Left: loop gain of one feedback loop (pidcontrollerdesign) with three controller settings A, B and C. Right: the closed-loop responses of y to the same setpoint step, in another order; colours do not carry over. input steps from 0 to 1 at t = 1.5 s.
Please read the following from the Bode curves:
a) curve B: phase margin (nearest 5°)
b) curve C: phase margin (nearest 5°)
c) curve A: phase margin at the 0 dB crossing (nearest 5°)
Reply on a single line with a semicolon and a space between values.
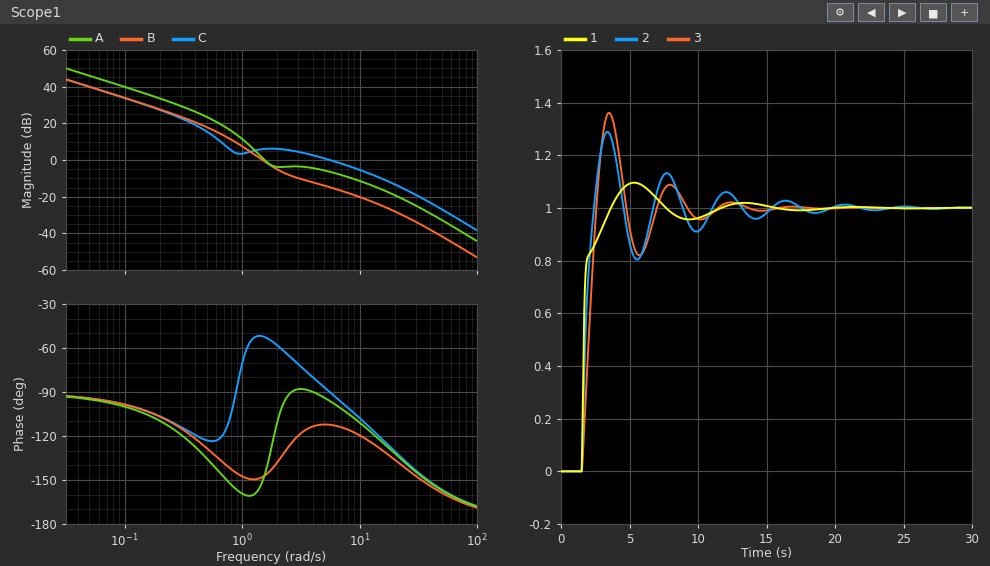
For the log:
30°; 90°; 35°
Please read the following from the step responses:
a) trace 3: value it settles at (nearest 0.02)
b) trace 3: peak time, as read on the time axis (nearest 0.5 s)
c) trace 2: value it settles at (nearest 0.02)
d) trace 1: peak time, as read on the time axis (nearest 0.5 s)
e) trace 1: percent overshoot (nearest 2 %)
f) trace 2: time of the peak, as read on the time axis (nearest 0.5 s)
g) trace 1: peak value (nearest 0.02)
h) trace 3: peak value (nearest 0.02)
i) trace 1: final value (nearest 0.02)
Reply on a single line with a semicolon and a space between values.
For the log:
1.00; 3.5 s; 1.00; 5.5 s; 10 %; 3.5 s; 1.10; 1.36; 1.00
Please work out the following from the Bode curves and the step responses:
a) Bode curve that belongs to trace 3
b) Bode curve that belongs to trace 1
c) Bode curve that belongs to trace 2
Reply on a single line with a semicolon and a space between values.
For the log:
B; C; A
